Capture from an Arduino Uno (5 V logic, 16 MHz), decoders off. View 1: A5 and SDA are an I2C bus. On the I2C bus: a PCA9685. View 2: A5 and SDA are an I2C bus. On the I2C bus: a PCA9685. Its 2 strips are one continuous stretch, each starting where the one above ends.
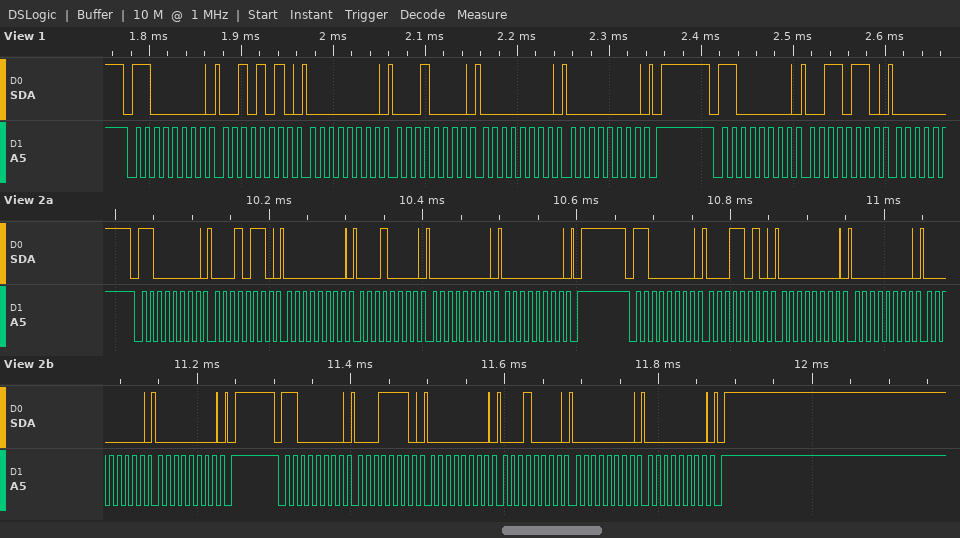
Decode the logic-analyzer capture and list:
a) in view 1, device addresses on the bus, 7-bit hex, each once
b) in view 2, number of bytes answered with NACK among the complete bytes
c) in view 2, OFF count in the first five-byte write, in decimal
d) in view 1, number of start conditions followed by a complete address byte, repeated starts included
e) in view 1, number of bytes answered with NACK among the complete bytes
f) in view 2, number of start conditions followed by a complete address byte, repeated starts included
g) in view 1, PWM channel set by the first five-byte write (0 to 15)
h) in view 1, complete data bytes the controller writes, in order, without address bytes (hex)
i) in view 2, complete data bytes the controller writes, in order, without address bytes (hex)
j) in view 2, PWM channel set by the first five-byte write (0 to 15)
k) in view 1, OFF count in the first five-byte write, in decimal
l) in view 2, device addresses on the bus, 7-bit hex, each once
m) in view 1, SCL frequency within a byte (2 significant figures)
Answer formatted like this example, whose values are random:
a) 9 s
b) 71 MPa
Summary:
a) 0x60
b) 0
c) 0
d) 2
e) 0
f) 3
g) 9
h) 2A 00 10 00 00 36
i) 16 00 10 00 00 1A 00 00 00 00 1E 00 10 00 00
j) 4
k) 0
l) 0x60
m) 100 kHz
